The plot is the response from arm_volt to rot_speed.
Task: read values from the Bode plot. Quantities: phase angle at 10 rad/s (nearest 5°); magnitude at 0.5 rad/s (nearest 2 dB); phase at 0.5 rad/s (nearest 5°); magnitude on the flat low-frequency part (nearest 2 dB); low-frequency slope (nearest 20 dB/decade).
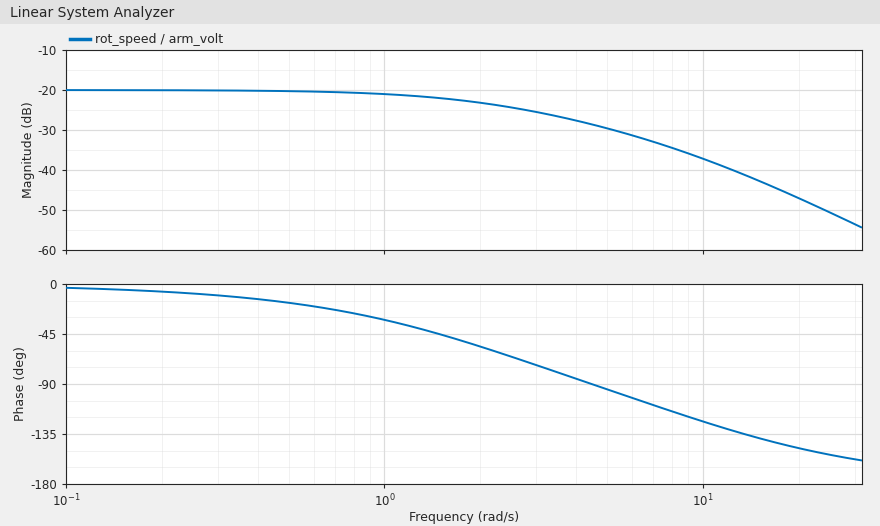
-125°
-20 dB
-15°
-20 dB
0 dB/decade
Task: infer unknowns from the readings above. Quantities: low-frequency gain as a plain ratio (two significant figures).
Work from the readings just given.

0.10
